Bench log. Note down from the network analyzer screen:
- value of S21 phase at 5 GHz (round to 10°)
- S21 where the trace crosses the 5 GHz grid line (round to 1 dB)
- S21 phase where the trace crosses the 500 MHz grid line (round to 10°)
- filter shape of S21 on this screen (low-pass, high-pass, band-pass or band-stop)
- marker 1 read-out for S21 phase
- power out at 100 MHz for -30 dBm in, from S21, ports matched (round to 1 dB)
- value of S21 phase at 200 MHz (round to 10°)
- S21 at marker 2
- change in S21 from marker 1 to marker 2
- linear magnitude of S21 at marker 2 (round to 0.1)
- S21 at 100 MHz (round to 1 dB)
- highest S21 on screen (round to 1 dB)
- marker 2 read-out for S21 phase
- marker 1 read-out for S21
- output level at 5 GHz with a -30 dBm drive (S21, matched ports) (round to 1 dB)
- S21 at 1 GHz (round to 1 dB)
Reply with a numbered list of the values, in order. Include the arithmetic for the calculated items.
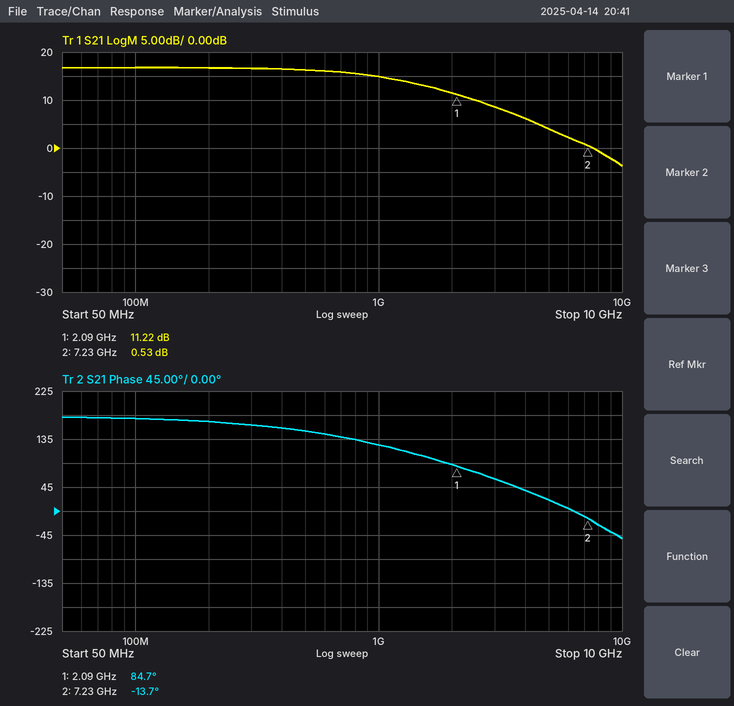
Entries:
1. 20°
2. 4 dB
3. 150°
4. low-pass
5. 84.7°
6. -30 dBm + (17 dB) = -13 dBm
7. 170°
8. 0.53 dB
9. 0.53 − (11.22) = -10.69 dB
10. 10^(0.53/20) ≈ 1.1
11. 17 dB
12. 17 dB
13. -13.7°
14. 11.22 dB
15. -30 dBm + (4 dB) = -26 dBm
16. 15 dB
